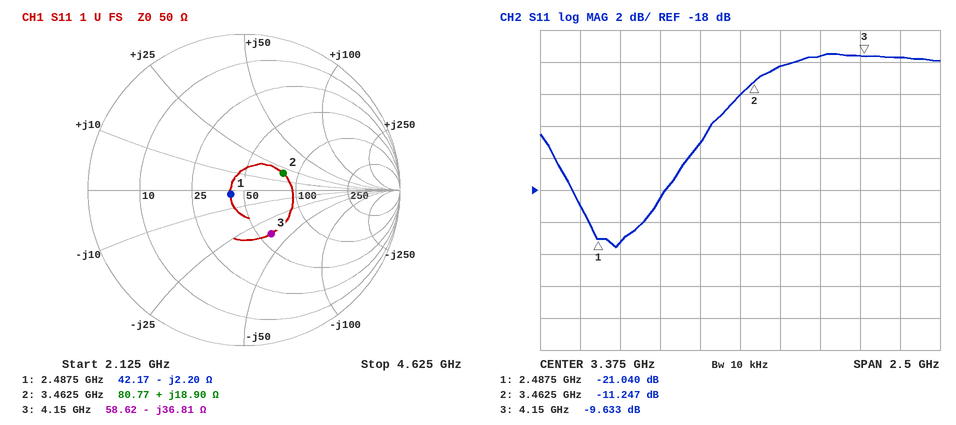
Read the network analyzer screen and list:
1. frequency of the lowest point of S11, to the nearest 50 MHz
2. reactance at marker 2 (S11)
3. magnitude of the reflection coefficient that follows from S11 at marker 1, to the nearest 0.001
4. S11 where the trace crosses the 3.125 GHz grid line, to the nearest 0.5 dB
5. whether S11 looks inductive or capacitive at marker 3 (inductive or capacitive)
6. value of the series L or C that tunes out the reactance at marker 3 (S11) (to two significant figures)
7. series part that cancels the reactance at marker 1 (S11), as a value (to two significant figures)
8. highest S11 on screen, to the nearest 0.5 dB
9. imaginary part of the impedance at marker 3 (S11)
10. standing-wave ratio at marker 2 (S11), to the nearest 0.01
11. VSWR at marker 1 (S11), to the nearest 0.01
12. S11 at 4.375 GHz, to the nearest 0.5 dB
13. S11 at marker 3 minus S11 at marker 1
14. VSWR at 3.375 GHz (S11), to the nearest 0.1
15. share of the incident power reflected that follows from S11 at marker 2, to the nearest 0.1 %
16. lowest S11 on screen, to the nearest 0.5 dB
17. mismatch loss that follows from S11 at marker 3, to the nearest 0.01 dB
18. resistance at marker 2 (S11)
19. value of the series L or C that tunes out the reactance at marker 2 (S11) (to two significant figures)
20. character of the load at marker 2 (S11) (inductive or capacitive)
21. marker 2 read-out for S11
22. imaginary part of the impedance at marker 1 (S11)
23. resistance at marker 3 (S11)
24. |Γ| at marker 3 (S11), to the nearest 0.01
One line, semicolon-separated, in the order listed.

2.60 GHz; +18.90 Ω; 0.089; -15.0 dB; capacitive; 1.4 nH; 140 pH; -9.5 dB; -36.81 Ω; 1.75; 1.19; -9.5 dB; 11.407 dB; 1.7; 7.5 %; -21.5 dB; 0.50 dB; 80.77 Ω; 2.4 pF; inductive; -11.247 dB; -2.20 Ω; 58.62 Ω; 0.33
